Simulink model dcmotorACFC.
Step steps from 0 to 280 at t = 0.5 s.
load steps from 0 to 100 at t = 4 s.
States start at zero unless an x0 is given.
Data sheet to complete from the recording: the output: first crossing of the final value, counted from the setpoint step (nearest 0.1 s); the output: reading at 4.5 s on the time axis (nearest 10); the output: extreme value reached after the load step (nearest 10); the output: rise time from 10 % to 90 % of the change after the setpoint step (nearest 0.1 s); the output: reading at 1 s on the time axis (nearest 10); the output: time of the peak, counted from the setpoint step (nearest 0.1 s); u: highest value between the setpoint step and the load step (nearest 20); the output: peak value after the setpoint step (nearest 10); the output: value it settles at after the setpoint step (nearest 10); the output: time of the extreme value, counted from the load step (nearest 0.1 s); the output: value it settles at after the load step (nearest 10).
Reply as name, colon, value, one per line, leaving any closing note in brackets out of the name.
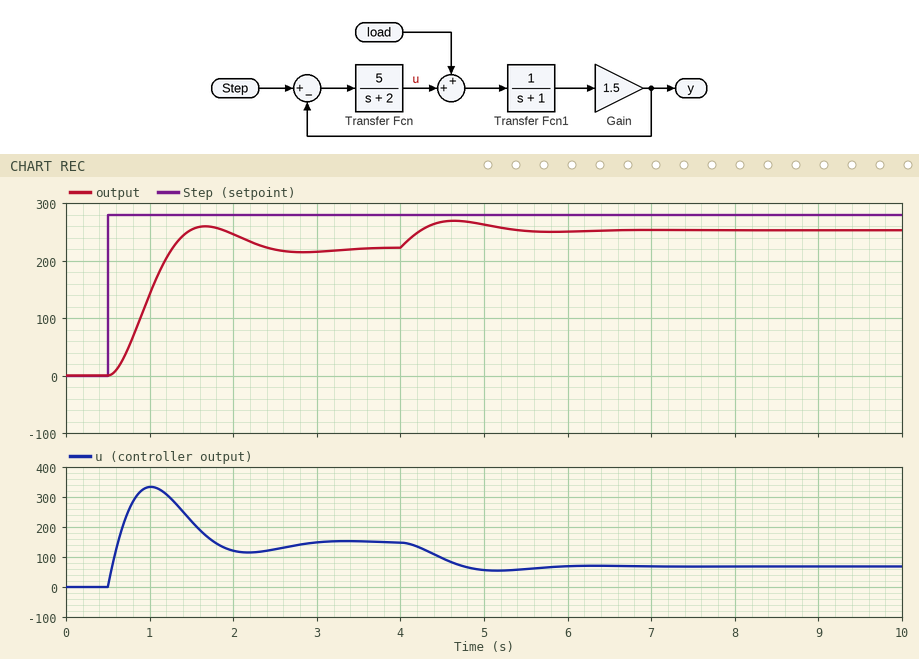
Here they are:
the output: first crossing of the final value, counted from the setpoint step: 0.8 s
the output: reading at 4.5 s on the time axis: 270
the output: extreme value reached after the load step: 270
the output: rise time from 10 % to 90 % of the change after the setpoint step: 0.5 s
the output: reading at 1 s on the time axis: 140
the output: time of the peak, counted from the setpoint step: 1.2 s
u: highest value between the setpoint step and the load step: 340
the output: peak value after the setpoint step: 260
the output: value it settles at after the setpoint step: 220
the output: time of the extreme value, counted from the load step: 0.6 s
the output: value it settles at after the load step: 250
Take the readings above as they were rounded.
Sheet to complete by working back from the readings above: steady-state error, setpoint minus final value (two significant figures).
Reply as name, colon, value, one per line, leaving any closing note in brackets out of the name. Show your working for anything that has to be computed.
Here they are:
steady-state error, setpoint minus final value: 280 - 220 = 60
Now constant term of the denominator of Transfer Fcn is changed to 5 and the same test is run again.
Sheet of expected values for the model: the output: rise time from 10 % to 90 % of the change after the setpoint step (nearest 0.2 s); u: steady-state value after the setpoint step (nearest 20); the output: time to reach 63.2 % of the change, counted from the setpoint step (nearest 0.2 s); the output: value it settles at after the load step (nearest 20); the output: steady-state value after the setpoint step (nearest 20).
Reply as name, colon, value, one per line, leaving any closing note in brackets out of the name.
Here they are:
the output: rise time from 10 % to 90 % of the change after the setpoint step: 0.8 s
u: steady-state value after the setpoint step: 120
the output: time to reach 63.2 % of the change, counted from the setpoint step: 0.6 s
the output: value it settles at after the load step: 220
the output: steady-state value after the setpoint step: 160
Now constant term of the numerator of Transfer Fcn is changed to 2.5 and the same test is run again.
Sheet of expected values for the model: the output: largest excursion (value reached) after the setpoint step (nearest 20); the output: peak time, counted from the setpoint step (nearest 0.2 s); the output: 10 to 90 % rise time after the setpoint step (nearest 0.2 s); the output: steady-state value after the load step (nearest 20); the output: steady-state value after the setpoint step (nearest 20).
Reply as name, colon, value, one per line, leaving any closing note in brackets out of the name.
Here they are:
the output: largest excursion (value reached) after the setpoint step: 200
the output: peak time, counted from the setpoint step: 1.6 s
the output: 10 to 90 % rise time after the setpoint step: 0.8 s
the output: steady-state value after the load step: 240
the output: steady-state value after the setpoint step: 180
